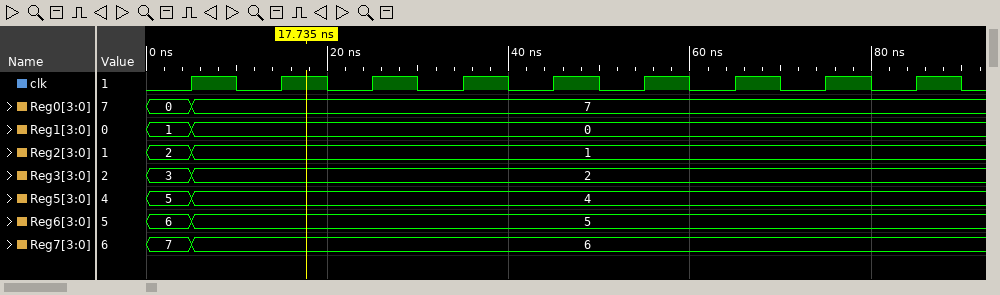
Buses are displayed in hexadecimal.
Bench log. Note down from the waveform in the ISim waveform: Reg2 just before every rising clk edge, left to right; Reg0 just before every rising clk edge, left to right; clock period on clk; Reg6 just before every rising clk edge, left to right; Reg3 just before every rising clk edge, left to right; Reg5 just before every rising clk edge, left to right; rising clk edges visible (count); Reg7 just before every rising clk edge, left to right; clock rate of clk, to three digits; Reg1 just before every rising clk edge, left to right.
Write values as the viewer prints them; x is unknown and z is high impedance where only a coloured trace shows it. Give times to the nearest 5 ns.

2, 1, 1, 1, 1, 1, 1, 1, 1
0, 7, 7, 7, 7, 7, 7, 7, 7
10 ns
6, 5, 5, 5, 5, 5, 5, 5, 5
3, 2, 2, 2, 2, 2, 2, 2, 2
5, 4, 4, 4, 4, 4, 4, 4, 4
9
7, 6, 6, 6, 6, 6, 6, 6, 6
100 MHz
1, 0, 0, 0, 0, 0, 0, 0, 0
